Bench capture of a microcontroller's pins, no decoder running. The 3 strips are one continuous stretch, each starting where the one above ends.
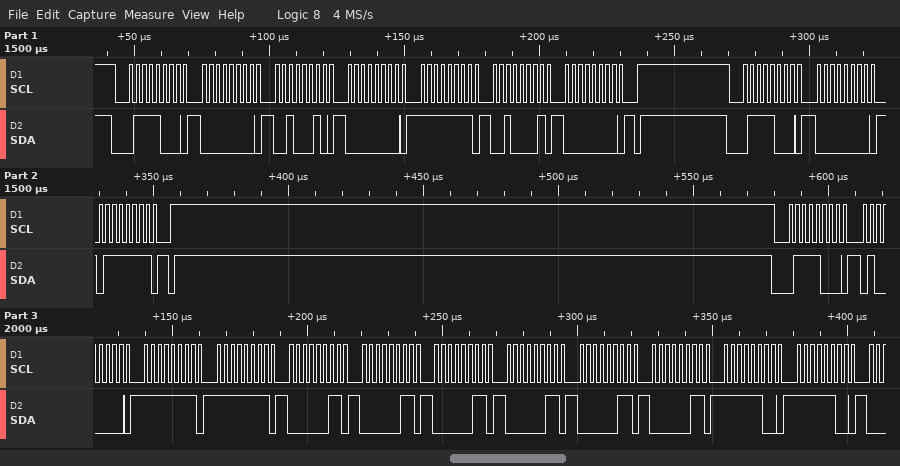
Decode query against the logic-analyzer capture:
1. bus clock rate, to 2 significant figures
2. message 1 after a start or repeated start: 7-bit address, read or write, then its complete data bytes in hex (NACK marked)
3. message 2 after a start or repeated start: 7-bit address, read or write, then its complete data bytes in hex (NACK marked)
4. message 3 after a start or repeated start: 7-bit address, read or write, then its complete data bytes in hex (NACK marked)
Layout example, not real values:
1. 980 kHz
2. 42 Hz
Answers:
1. 400 kHz
2. 0x3C write: 00 22 00 FF 21 00
3. 0x3C write: 00 7F
4. 0x3C write: 40 FF FF 03 03 03 03 03 03 FC FC
